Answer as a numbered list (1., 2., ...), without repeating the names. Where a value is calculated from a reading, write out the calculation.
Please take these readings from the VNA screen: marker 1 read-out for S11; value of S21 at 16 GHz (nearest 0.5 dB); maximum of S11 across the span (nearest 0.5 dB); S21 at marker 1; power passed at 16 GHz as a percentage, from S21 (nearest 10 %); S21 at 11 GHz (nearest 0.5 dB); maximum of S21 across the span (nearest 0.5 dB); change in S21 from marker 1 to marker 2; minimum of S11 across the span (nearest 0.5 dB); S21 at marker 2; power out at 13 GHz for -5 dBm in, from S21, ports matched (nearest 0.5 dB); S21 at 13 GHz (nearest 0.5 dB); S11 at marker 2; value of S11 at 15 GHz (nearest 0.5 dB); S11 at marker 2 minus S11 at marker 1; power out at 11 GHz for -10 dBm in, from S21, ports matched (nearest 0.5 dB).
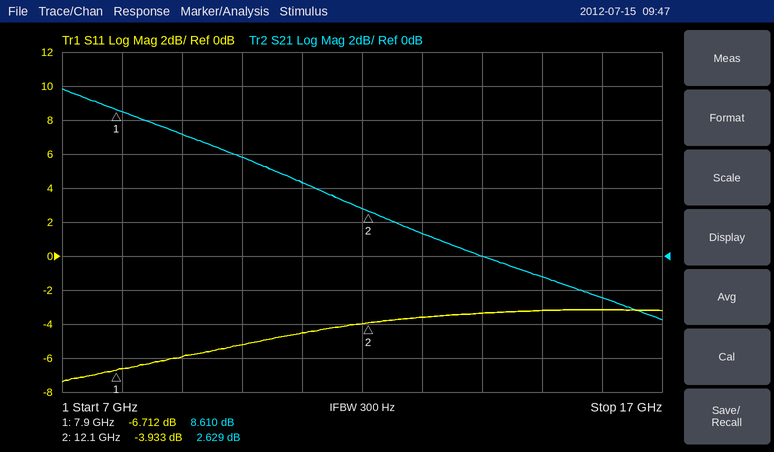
1. -6.712 dB
2. -2.5 dB
3. -3.0 dB
4. 8.610 dB
5. 10^(-2.5/10) ≈ 56.2 %, so 60 % to the nearest 10 %
6. 4.5 dB
7. 10.0 dB
8. 2.629 − (8.61) = -5.981 dB
9. -7.5 dB
10. 2.629 dB
11. -5 dBm + (1.5 dB) = -3.5 dBm
12. 1.5 dB
13. -3.933 dB
14. -3.0 dB
15. -3.933 − (-6.712) = 2.779 dB
16. -10 dBm + (4.5 dB) = -5.5 dBm
